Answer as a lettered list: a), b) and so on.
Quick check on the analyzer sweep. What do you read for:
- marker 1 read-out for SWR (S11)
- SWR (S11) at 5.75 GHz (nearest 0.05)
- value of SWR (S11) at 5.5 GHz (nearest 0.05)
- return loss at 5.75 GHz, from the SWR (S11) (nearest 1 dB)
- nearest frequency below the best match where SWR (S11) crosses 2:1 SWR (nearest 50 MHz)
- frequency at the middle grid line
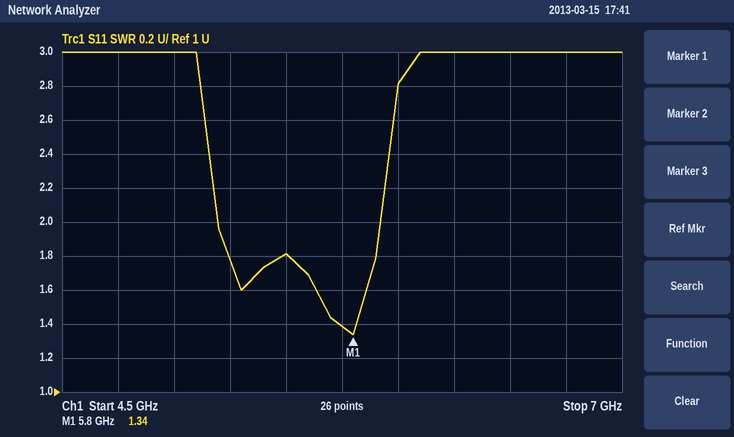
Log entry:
a) 1.34
b) 1.40
c) 1.80
d) 16 dB
e) 5.20 GHz
f) 5.75 GHz
